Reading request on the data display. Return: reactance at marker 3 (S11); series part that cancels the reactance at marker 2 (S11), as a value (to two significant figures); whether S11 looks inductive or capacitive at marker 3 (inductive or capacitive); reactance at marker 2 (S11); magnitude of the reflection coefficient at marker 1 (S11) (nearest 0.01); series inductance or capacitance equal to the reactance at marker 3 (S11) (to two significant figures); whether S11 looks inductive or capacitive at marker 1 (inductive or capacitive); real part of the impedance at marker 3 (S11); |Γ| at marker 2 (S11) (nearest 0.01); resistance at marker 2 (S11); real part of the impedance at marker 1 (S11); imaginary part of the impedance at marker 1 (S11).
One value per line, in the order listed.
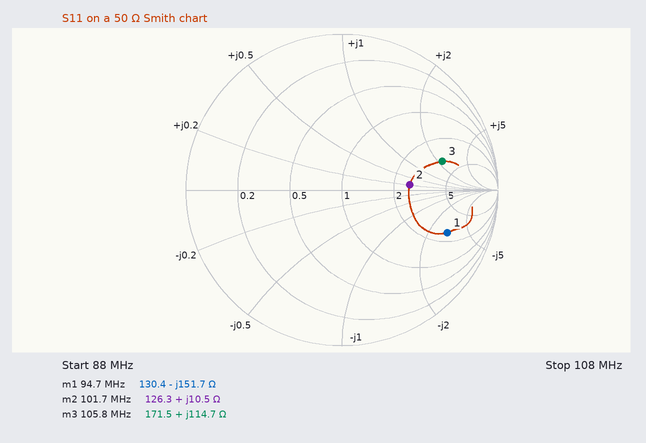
+114.7 Ω
150 pF
inductive
+10.5 Ω
0.73
170 nH
capacitive
171.5 Ω
0.44
126.3 Ω
130.4 Ω
-151.7 Ω
